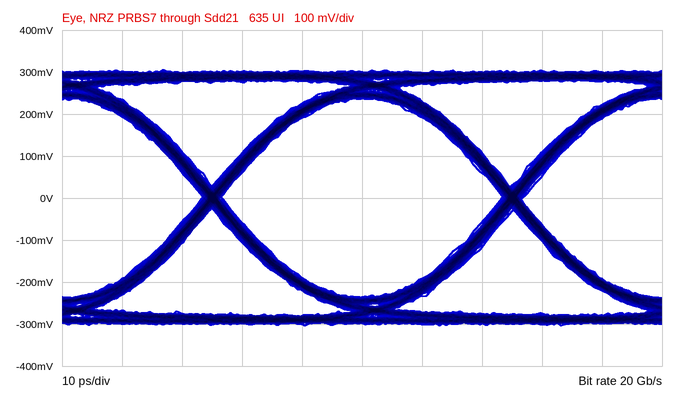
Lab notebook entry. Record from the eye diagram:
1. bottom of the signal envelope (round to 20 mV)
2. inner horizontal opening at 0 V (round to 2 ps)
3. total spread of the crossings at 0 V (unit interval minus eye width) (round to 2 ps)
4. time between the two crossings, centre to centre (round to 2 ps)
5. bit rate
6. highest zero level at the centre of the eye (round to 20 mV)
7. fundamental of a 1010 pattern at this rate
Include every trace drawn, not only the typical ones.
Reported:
-300 mV
46 ps
4 ps
50 ps
20 Gb/s
-240 mV
10 GHz
